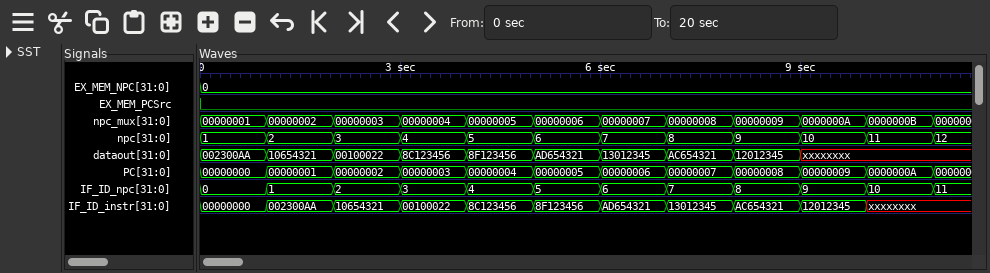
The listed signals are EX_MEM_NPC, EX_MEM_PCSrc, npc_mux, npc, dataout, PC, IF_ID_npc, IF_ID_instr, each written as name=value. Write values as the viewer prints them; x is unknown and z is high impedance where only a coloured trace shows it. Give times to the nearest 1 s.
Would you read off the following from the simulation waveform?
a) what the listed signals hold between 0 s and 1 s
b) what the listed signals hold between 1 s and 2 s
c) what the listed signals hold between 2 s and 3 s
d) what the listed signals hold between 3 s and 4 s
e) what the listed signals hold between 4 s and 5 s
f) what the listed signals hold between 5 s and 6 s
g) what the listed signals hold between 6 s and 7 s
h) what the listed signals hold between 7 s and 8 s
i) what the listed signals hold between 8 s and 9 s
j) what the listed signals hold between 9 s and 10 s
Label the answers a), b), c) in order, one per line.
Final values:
a) EX_MEM_NPC=0, EX_MEM_PCSrc=0, npc_mux=00000001, npc=1, dataout=002300AA, PC=00000000, IF_ID_npc=0, IF_ID_instr=00000000
b) EX_MEM_NPC=0, EX_MEM_PCSrc=0, npc_mux=00000002, npc=2, dataout=10654321, PC=00000001, IF_ID_npc=1, IF_ID_instr=002300AA
c) EX_MEM_NPC=0, EX_MEM_PCSrc=0, npc_mux=00000003, npc=3, dataout=00100022, PC=00000002, IF_ID_npc=2, IF_ID_instr=10654321
d) EX_MEM_NPC=0, EX_MEM_PCSrc=0, npc_mux=00000004, npc=4, dataout=8C123456, PC=00000003, IF_ID_npc=3, IF_ID_instr=00100022
e) EX_MEM_NPC=0, EX_MEM_PCSrc=0, npc_mux=00000005, npc=5, dataout=8F123456, PC=00000004, IF_ID_npc=4, IF_ID_instr=8C123456
f) EX_MEM_NPC=0, EX_MEM_PCSrc=0, npc_mux=00000006, npc=6, dataout=AD654321, PC=00000005, IF_ID_npc=5, IF_ID_instr=8F123456
g) EX_MEM_NPC=0, EX_MEM_PCSrc=0, npc_mux=00000007, npc=7, dataout=13012345, PC=00000006, IF_ID_npc=6, IF_ID_instr=AD654321
h) EX_MEM_NPC=0, EX_MEM_PCSrc=0, npc_mux=00000008, npc=8, dataout=AC654321, PC=00000007, IF_ID_npc=7, IF_ID_instr=13012345
i) EX_MEM_NPC=0, EX_MEM_PCSrc=0, npc_mux=00000009, npc=9, dataout=12012345, PC=00000008, IF_ID_npc=8, IF_ID_instr=AC654321
j) EX_MEM_NPC=0, EX_MEM_PCSrc=0, npc_mux=0000000A, npc=10, dataout=xxxxxxxx, PC=00000009, IF_ID_npc=9, IF_ID_instr=12012345
